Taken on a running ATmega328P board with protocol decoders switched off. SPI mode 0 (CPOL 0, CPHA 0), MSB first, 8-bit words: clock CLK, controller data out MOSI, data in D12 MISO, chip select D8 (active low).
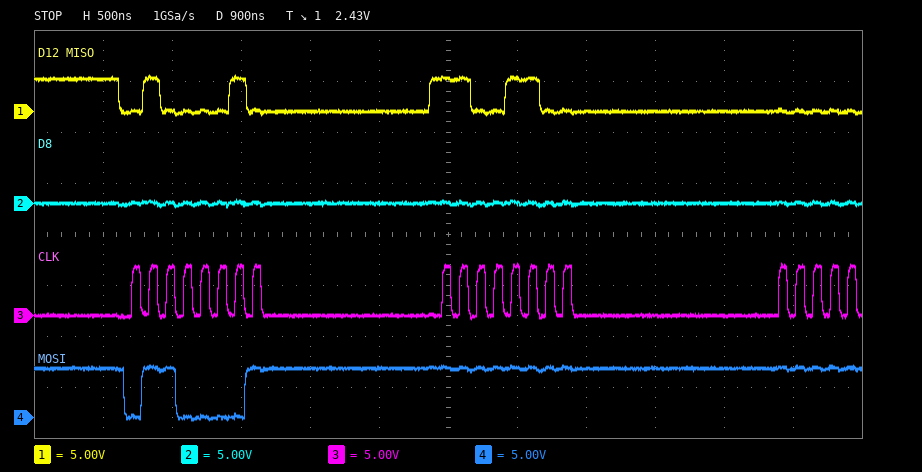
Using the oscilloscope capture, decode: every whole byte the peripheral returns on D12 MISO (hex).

0x42 0xCC
